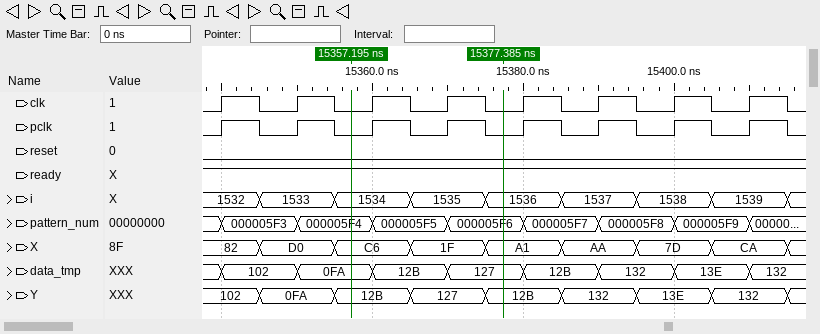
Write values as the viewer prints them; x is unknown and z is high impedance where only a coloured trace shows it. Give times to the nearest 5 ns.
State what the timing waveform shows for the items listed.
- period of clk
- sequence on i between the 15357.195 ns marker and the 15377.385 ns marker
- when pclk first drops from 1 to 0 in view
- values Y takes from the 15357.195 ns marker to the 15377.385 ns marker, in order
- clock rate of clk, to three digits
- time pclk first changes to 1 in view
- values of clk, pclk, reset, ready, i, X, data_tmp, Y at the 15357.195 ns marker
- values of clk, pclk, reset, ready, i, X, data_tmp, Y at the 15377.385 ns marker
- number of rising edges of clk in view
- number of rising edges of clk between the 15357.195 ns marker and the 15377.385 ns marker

10 ns
1534, 1535, 1536
15345 ns
12B, 127, 12B
100 MHz
15340 ns
clk=0, pclk=0, reset=0, ready=1, i=1534, X=C6, data_tmp=0FA, Y=12B
clk=0, pclk=0, reset=0, ready=1, i=1536, X=A1, data_tmp=127, Y=12B
8
2
